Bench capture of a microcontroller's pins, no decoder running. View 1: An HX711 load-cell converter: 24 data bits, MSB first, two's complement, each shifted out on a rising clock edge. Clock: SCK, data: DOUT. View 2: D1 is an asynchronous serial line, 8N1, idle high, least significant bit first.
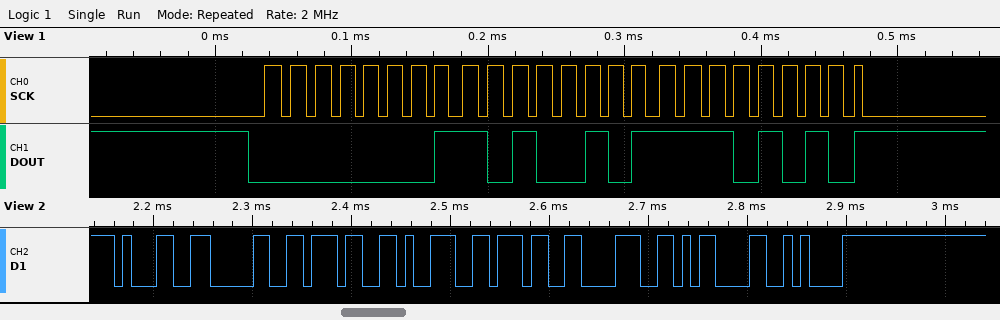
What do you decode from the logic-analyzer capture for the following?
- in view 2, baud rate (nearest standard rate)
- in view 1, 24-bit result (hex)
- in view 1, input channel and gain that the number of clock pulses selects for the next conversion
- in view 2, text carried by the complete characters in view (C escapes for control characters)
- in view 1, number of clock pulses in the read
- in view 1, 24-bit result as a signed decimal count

115200 baud
0x01A5EA
channel A, gain 128
"107978\r\n"
25
108010
